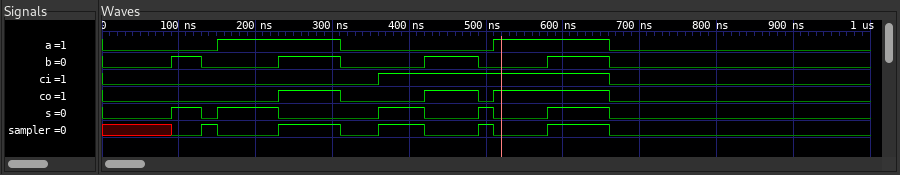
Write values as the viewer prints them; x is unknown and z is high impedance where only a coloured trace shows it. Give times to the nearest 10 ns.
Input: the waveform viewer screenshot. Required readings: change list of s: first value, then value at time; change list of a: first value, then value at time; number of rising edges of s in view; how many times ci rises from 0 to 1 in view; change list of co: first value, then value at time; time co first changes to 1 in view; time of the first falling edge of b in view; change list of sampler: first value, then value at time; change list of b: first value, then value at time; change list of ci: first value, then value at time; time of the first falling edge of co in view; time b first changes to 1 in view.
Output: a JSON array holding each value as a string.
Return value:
["0, 1 at 90 ns, 0 at 130 ns, 1 at 150 ns, 0 at 230 ns, 1 at 360 ns, 0 at 420 ns, 1 at 490 ns, 0 at 510 ns, 1 at 580 ns, 0 at 660 ns", "0, 1 at 150 ns, 0 at 310 ns, 1 at 510 ns, 0 at 660 ns", "5", "1", "0, 1 at 230 ns, 0 at 310 ns, 1 at 420 ns, 0 at 490 ns, 1 at 510 ns, 0 at 660 ns", "230 ns", "130 ns", "x, 0 at 90 ns, 1 at 130 ns, 0 at 150 ns, 1 at 230 ns, 0 at 310 ns, 1 at 360 ns, 0 at 420 ns, 1 at 490 ns, 0 at 510 ns, 1 at 580 ns, 0 at 660 ns", "0, 1 at 90 ns, 0 at 130 ns, 1 at 230 ns, 0 at 310 ns, 1 at 420 ns, 0 at 490 ns, 1 at 580 ns, 0 at 660 ns", "0, 1 at 360 ns, 0 at 660 ns", "310 ns", "90 ns"]
